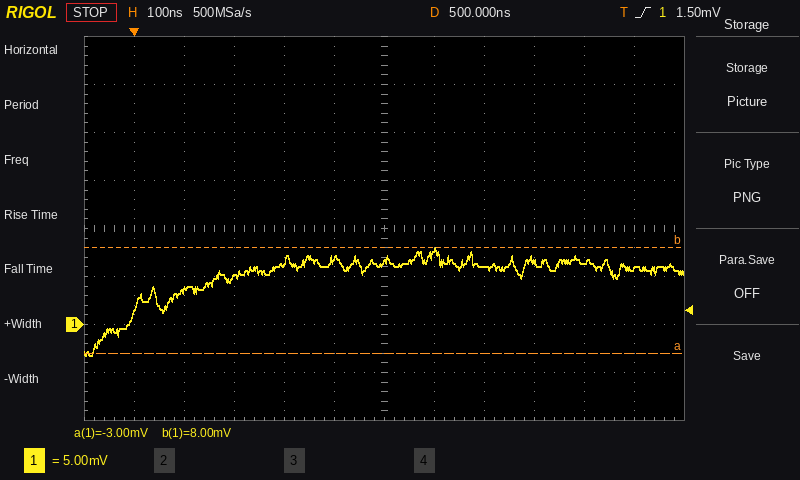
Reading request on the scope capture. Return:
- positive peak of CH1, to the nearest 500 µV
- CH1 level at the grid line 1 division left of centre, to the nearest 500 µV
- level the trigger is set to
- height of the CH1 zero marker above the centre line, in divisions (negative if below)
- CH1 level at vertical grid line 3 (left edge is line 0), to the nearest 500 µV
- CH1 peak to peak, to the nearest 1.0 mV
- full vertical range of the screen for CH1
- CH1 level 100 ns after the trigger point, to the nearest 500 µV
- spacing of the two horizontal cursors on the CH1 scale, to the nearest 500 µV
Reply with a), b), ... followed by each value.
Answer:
a) 8.0 mV
b) 7.0 mV
c) 1.50 mV
d) -2.0 div
e) 5.0 mV
f) 11.0 mV
g) 40 mV
h) 3.5 mV
i) 11.0 mV
